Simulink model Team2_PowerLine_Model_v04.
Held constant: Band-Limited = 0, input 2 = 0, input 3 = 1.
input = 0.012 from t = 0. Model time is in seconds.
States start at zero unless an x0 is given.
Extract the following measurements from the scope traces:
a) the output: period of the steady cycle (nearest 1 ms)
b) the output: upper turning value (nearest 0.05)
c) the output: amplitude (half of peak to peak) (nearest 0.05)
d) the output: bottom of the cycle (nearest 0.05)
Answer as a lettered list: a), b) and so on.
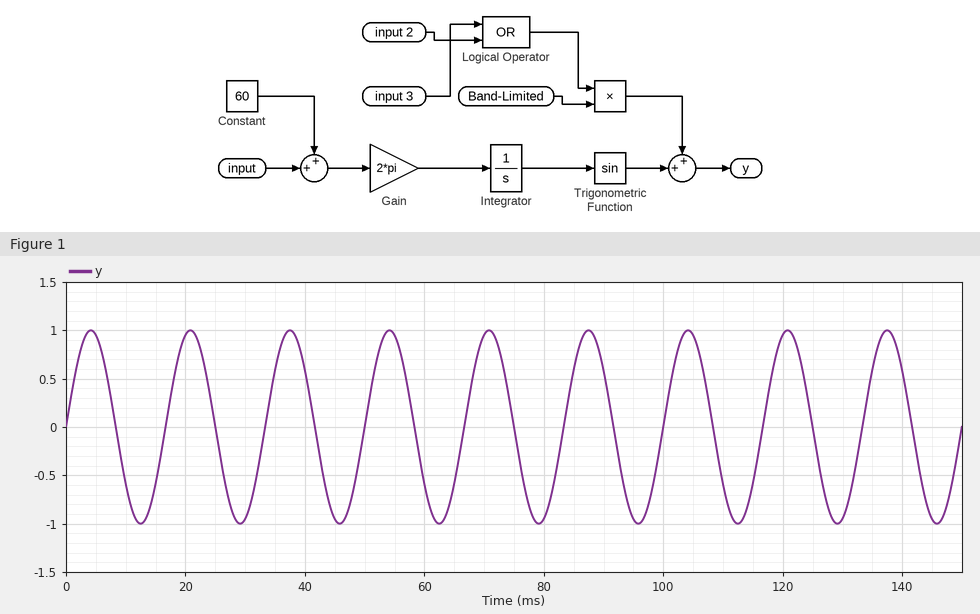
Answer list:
a) 17 ms
b) 1.00
c) 1.00
d) -1.00
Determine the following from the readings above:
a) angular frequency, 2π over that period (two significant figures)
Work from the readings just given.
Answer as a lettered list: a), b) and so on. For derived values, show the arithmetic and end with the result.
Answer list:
a) 2π / 17 = 0.37 rad/ms
